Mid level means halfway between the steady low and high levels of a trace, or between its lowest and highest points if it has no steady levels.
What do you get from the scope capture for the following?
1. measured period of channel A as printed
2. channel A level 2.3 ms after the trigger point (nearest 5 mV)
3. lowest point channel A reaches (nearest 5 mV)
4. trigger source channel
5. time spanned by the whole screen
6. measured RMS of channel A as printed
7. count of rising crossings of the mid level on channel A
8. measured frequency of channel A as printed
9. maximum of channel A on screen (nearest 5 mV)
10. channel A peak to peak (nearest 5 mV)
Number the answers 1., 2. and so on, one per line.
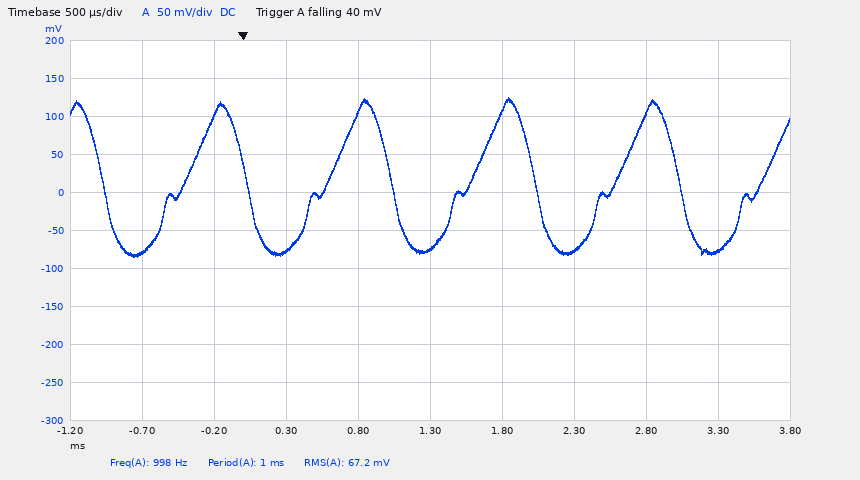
1. 1 ms
2. -75 mV
3. -85 mV
4. channel A
5. 5 ms
6. 67.2 mV
7. 5
8. 998 Hz
9. 125 mV
10. 210 mV
